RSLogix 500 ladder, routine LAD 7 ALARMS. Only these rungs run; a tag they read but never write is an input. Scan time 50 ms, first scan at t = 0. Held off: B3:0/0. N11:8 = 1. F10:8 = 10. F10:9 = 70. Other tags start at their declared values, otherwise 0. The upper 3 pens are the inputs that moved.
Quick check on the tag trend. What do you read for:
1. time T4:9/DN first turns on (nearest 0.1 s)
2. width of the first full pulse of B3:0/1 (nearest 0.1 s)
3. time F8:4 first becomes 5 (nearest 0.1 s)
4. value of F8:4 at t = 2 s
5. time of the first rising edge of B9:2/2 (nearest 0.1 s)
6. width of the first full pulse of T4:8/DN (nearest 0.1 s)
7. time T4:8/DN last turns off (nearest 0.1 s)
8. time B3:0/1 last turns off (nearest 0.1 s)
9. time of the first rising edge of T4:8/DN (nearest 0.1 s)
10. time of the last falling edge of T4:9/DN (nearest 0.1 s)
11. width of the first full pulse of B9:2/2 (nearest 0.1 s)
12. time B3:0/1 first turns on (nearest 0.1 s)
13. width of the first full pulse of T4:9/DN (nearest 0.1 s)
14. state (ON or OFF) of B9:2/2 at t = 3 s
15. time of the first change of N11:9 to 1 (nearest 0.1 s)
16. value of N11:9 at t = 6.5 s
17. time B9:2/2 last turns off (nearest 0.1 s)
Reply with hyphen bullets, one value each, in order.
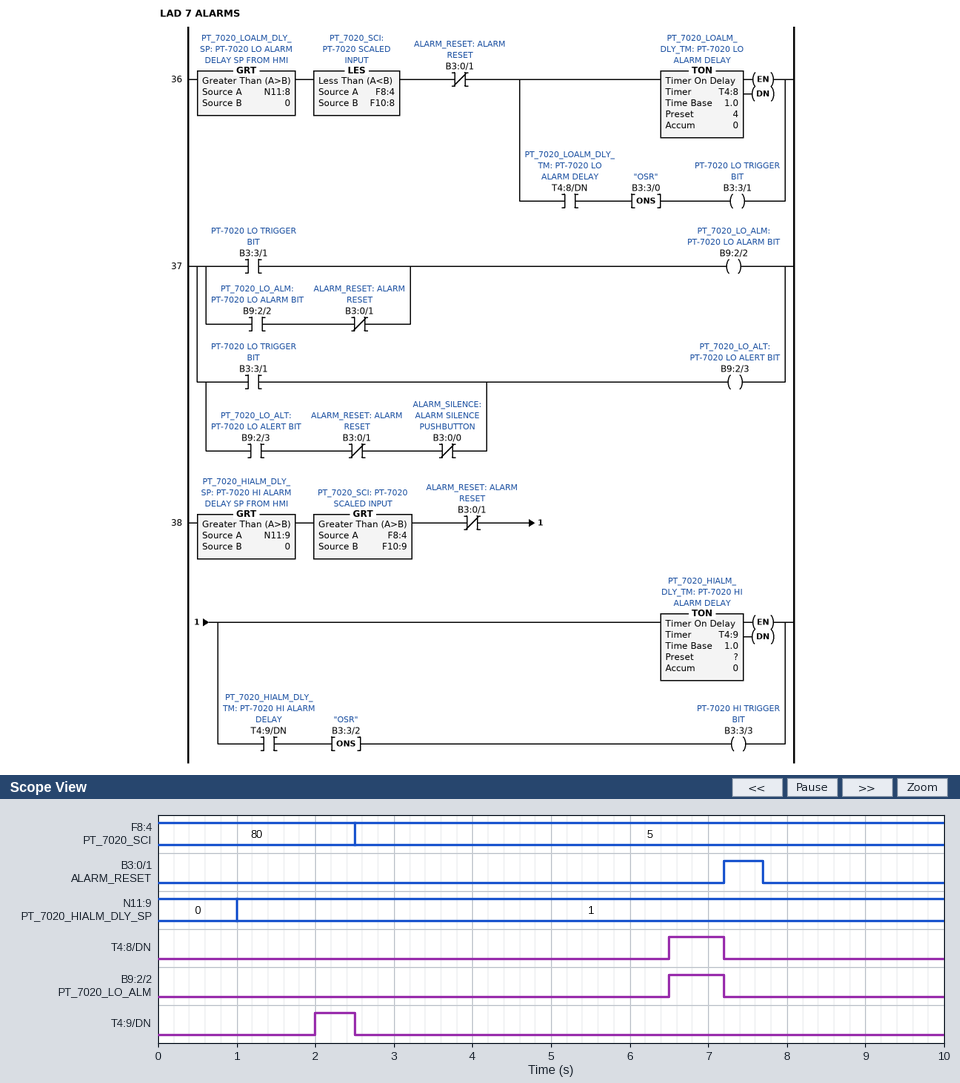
- 2.0 s
- 0.5 s
- 2.5 s
- 80
- 6.5 s
- 0.7 s
- 7.2 s
- 7.7 s
- 6.5 s
- 2.5 s
- 0.7 s
- 7.2 s
- 0.5 s
- OFF
- 1.0 s
- 1
- 7.2 s
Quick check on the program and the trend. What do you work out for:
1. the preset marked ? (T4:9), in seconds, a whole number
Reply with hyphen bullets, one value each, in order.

- 1 s
